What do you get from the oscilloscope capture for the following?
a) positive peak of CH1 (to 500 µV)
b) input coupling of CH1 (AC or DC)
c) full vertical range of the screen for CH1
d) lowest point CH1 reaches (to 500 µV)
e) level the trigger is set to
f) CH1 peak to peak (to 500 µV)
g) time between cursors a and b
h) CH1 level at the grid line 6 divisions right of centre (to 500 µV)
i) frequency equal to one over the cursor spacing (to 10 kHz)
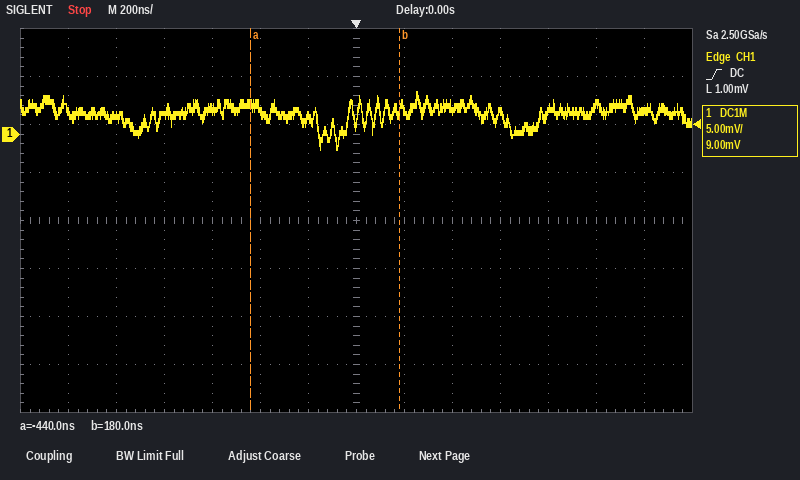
4.5 mV
DC
40 mV
-1.5 mV
1.00 mV
6.0 mV
620 ns
2.5 mV
1.61 MHz
